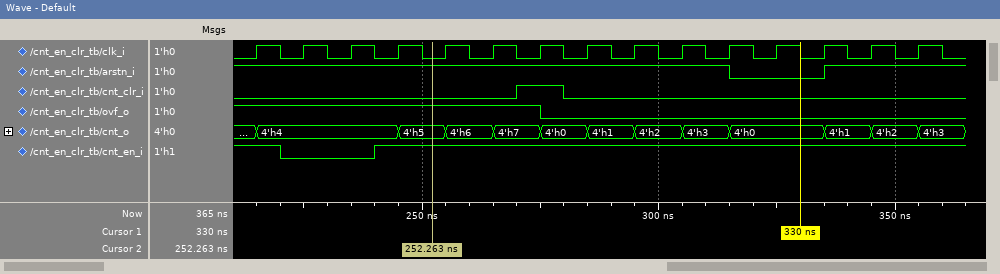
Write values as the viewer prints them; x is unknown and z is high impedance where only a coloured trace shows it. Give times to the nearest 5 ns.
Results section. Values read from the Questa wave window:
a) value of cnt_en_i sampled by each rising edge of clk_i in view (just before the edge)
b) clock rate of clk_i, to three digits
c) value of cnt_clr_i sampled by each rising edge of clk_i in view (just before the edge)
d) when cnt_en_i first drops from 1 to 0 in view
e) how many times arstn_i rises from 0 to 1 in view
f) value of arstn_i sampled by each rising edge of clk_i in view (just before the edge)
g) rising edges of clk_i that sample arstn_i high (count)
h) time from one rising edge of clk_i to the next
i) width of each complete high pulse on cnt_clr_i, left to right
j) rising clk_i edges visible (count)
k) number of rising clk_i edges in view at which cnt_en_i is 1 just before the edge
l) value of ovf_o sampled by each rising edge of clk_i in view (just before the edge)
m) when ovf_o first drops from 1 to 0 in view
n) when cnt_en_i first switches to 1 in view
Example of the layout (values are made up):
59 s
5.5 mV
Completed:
1 0 0 1 1 1 1 1 1 1 1 1 1 1 1
100 MHz
0 0 0 0 0 0 1 0 0 0 0 0 0 0 0
220 ns
1
1 1 1 1 1 1 1 1 1 1 1 0 0 1 1
13
10 ns
10 ns
15
13
1 1 1 1 1 1 1 0 0 0 0 0 0 0 0
275 ns
240 ns
